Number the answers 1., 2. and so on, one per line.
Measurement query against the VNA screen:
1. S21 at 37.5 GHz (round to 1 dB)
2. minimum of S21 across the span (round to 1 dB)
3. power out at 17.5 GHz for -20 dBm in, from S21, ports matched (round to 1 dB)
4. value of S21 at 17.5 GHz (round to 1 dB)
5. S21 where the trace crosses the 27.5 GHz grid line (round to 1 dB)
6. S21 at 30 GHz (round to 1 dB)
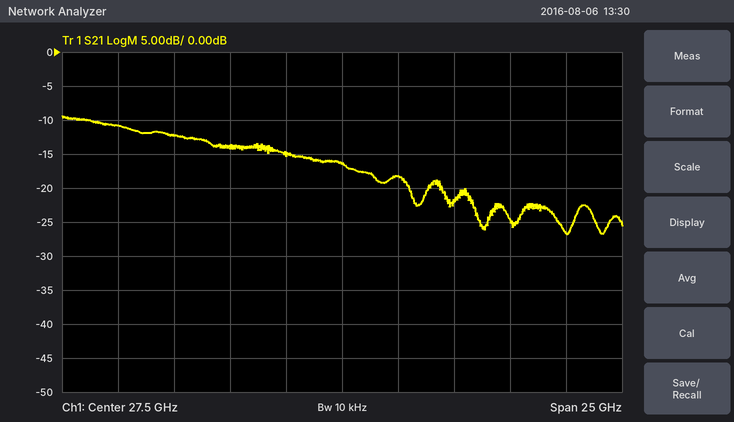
1. -27 dB
2. -27 dB
3. -31 dBm
4. -11 dB
5. -16 dB
6. -18 dB
